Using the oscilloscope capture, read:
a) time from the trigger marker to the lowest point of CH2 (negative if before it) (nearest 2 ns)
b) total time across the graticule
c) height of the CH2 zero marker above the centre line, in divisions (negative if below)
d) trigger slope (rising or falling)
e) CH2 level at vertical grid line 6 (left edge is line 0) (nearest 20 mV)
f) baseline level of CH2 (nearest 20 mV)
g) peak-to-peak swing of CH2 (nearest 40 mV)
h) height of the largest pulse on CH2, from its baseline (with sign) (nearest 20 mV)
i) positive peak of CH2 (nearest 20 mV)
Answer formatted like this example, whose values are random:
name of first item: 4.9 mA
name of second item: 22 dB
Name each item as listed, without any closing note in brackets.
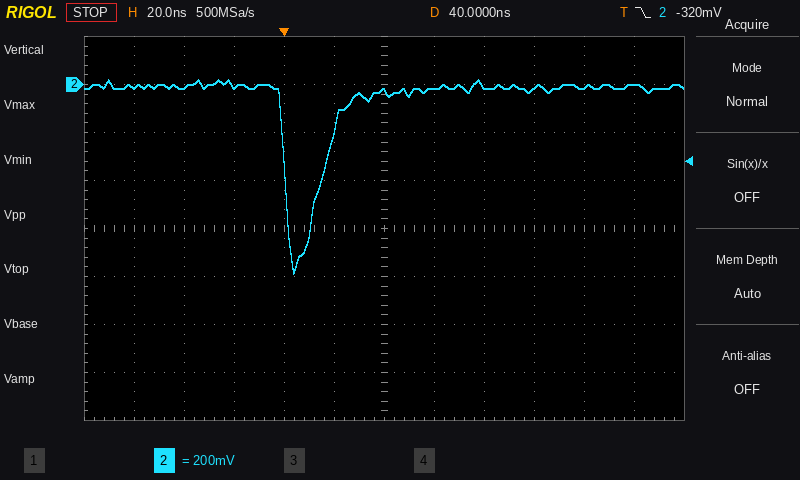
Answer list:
time from the trigger marker to the lowest point of CH2 (negative if before it): +4 ns
total time across the graticule: 240 ns
height of the CH2 zero marker above the centre line, in divisions: +3.0 div
trigger slope: falling
CH2 level at vertical grid line 6 (left edge is line 0): -20 mV
baseline level of CH2: -20 mV
peak-to-peak swing of CH2: 800 mV
height of the largest pulse on CH2, from its baseline (with sign): -780 mV
positive peak of CH2: 20 mV
